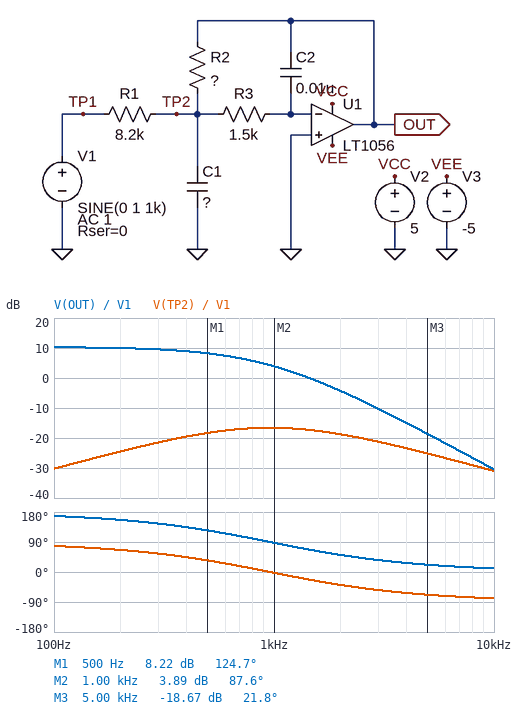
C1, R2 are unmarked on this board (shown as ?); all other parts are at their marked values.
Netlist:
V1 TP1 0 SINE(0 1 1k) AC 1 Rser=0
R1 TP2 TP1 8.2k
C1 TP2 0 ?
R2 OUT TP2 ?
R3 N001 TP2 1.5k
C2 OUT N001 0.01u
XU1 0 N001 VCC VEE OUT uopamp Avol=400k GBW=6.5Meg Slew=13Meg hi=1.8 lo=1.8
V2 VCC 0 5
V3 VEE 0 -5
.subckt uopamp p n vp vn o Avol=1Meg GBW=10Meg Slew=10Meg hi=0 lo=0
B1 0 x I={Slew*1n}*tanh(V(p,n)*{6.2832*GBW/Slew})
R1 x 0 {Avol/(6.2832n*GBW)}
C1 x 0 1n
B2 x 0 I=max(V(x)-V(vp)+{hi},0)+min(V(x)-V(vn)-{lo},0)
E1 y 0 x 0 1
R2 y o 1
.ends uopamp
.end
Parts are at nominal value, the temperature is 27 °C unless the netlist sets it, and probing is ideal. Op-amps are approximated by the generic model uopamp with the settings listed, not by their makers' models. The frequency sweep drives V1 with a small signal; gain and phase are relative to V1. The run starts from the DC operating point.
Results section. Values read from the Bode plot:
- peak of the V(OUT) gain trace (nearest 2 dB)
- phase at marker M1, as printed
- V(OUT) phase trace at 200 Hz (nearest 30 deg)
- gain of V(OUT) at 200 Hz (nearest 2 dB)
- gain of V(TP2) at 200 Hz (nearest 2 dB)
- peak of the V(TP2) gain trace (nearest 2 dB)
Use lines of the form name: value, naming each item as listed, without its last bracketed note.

peak of the V(OUT) gain trace: 10 dB
phase at marker M1, as printed: 124.7 deg
V(OUT) phase trace at 200 Hz: 150 deg
gain of V(OUT) at 200 Hz: 10 dB
gain of V(TP2) at 200 Hz: -24 dB
peak of the V(TP2) gain trace: -16 dB
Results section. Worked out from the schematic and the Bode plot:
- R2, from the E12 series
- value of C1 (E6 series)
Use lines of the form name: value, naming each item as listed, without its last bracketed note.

R2, from the E12 series: 27 kΩ
value of C1: 68 nF
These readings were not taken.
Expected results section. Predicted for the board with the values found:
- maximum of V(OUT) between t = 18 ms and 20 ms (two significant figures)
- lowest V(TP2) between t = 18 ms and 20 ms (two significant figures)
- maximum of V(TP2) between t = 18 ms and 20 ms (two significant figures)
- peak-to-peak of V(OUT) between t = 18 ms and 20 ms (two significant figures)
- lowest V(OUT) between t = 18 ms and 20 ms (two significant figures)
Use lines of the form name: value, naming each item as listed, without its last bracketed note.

maximum of V(OUT) between t = 18 ms and 20 ms: 1.6 V
lowest V(TP2) between t = 18 ms and 20 ms: -150 mV
maximum of V(TP2) between t = 18 ms and 20 ms: 150 mV
peak-to-peak of V(OUT) between t = 18 ms and 20 ms: 3.1 V
lowest V(OUT) between t = 18 ms and 20 ms: -1.6 V
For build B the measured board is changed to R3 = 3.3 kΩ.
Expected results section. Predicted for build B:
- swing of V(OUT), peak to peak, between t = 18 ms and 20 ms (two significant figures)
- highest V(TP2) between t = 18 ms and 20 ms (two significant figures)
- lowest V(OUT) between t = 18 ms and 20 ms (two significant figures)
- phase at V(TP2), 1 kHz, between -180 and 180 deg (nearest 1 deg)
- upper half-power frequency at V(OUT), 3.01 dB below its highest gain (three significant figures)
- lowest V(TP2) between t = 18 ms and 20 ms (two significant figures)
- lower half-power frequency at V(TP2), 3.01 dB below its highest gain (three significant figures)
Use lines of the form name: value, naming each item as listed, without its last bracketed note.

swing of V(OUT), peak to peak, between t = 18 ms and 20 ms: 2.2 V
highest V(TP2) between t = 18 ms and 20 ms: 230 mV
lowest V(OUT) between t = 18 ms and 20 ms: -1.1 V
phase at V(TP2), 1 kHz, between -180 and 180 deg: -28 deg
upper half-power frequency at V(OUT), 3.01 dB below its highest gain: 532 Hz
lowest V(TP2) between t = 18 ms and 20 ms: -230 mV
lower half-power frequency at V(TP2), 3.01 dB below its highest gain: 302 Hz
